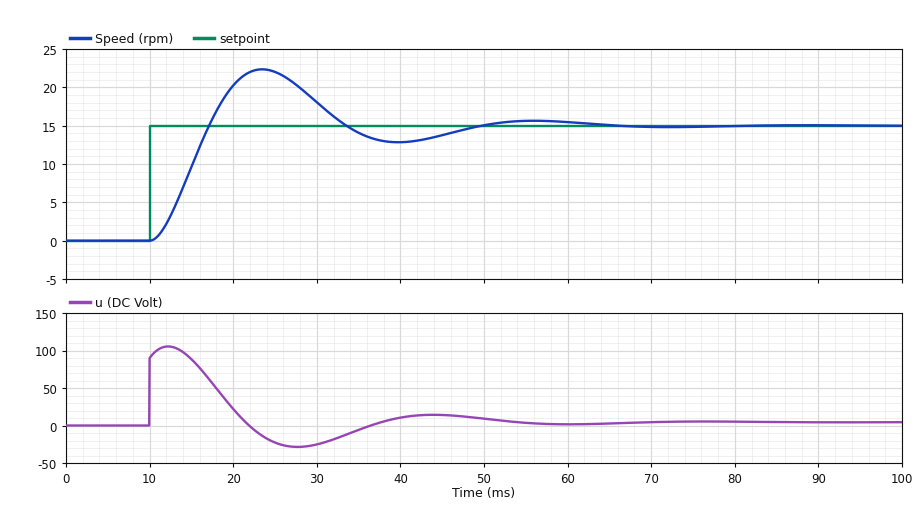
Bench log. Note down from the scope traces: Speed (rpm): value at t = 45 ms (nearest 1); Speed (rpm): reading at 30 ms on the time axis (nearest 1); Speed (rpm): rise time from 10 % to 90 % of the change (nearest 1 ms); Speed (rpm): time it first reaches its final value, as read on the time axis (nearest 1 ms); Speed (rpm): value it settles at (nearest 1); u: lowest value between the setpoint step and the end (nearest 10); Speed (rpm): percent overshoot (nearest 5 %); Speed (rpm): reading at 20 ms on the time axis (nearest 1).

14
18
5 ms
17 ms
15
-30
50 %
20
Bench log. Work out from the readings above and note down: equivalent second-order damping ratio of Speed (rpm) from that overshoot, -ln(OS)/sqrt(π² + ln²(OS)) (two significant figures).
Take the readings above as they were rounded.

0.22
